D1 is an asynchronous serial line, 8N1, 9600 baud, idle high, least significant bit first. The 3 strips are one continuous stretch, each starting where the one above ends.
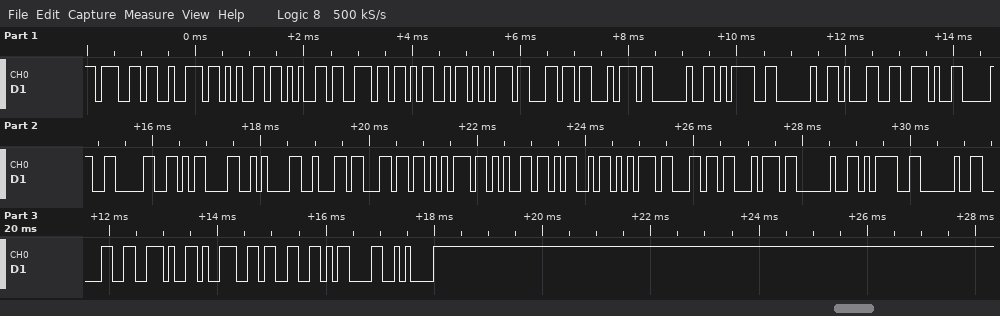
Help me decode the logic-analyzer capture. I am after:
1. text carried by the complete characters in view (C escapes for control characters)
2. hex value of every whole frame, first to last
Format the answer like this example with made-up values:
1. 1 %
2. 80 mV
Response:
1. "greenMult = 1.00\r\nblueMult = 0.93\r\n"
2. 67 72 65 65 6E 4D 75 6C 74 20 3D 20 31 2E 30 30 0D 0A 62 6C 75 65 4D 75 6C 74 20 3D 20 30 2E 39 33 0D 0A
